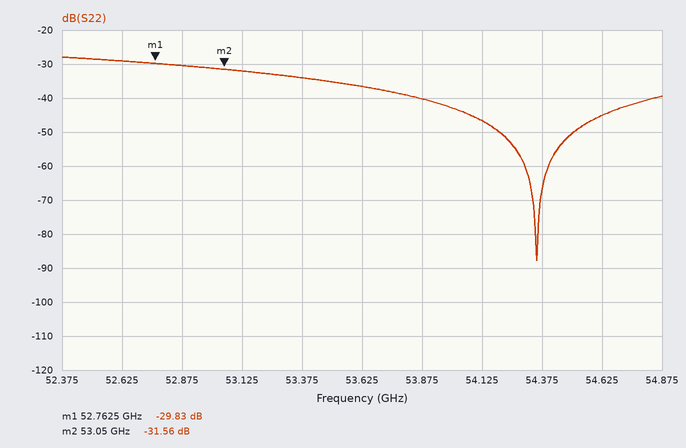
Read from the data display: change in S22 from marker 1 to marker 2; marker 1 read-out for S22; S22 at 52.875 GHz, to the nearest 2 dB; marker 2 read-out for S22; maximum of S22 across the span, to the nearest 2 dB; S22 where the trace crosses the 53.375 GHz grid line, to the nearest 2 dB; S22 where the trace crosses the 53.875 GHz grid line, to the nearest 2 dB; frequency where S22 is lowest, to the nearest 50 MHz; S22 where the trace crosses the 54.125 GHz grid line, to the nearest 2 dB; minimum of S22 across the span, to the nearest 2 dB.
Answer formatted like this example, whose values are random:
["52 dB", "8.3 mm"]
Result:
["-1.73 dB", "-29.83 dB", "-30 dB", "-31.56 dB", "-28 dB", "-34 dB", "-40 dB", "54.35 GHz", "-46 dB", "-88 dB"]
